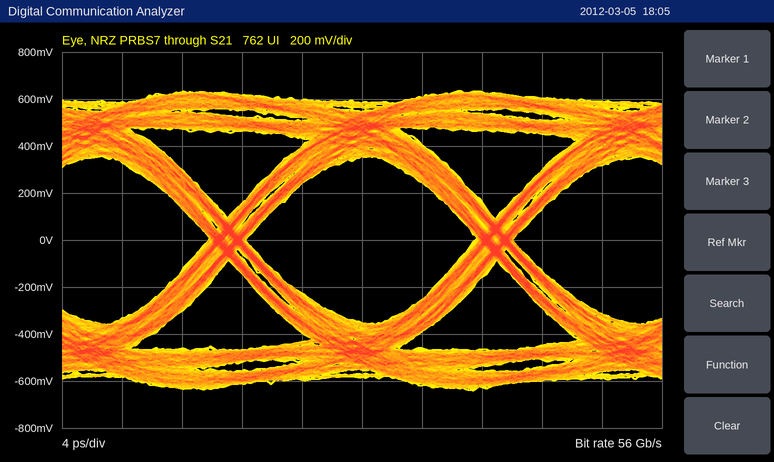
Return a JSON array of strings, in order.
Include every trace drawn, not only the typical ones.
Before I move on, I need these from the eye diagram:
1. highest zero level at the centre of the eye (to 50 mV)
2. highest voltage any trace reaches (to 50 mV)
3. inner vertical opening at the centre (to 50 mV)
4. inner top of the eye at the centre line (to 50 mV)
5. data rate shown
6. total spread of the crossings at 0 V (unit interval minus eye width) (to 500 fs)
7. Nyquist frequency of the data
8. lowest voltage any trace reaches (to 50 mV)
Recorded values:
["-350 mV", "650 mV", "700 mV", "350 mV", "56 Gb/s", "2.5 ps", "28 GHz", "-650 mV"]
